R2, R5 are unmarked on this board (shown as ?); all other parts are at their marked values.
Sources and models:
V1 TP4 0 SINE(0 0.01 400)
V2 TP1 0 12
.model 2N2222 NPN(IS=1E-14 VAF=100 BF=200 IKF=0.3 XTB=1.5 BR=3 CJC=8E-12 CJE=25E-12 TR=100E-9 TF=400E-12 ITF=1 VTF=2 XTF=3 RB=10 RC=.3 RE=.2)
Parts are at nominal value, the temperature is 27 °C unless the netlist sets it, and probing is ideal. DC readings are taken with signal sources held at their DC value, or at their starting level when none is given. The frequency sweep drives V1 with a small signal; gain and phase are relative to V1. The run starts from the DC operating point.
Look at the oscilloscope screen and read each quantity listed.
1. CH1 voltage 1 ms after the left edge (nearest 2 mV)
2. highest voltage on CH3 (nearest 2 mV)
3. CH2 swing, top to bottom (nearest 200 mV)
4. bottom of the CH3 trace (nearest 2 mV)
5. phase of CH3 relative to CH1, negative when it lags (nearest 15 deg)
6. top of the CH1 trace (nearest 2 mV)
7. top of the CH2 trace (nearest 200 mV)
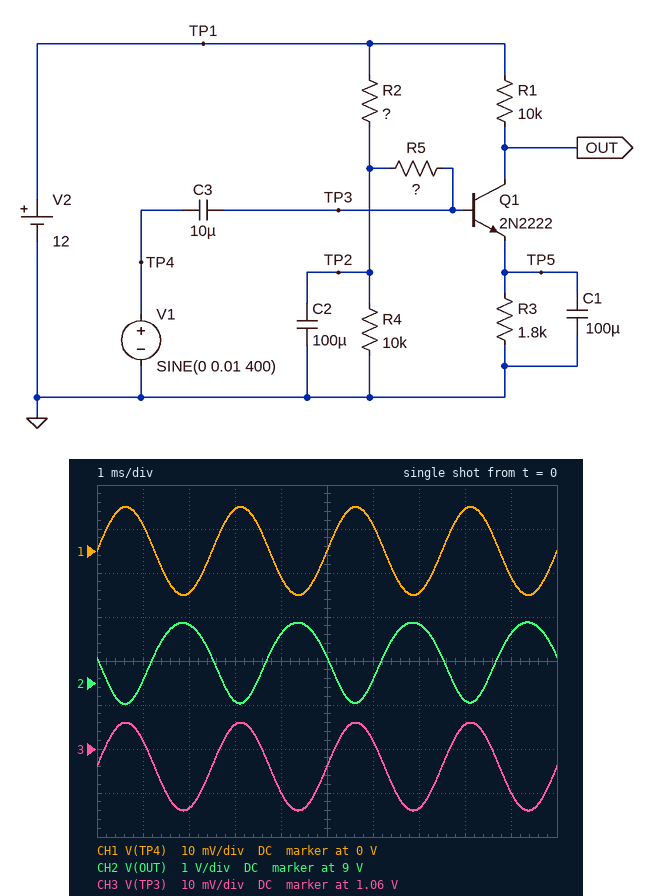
6 mV
1.066 V
1.8 V
1.046 V
0 deg
10 mV
10.4 V
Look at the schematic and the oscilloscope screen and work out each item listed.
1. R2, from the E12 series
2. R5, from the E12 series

100 kΩ
22 kΩ
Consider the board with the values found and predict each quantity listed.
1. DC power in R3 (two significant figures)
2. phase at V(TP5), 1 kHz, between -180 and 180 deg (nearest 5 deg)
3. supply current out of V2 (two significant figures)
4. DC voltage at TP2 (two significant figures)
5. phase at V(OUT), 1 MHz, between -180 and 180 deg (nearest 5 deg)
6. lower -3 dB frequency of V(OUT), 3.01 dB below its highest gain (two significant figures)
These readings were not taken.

110 µW
-90 deg
350 µA
1.1 V
165 deg
16 Hz
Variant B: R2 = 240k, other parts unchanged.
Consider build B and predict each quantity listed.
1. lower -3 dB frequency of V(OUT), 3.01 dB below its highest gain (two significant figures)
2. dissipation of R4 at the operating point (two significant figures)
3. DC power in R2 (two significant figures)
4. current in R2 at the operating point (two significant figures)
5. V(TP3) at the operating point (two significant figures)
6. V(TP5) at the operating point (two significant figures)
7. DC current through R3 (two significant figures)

3.7 MHz
23 µW
550 µW
48 µA
480 mV
2.1 mV
1.2 µA
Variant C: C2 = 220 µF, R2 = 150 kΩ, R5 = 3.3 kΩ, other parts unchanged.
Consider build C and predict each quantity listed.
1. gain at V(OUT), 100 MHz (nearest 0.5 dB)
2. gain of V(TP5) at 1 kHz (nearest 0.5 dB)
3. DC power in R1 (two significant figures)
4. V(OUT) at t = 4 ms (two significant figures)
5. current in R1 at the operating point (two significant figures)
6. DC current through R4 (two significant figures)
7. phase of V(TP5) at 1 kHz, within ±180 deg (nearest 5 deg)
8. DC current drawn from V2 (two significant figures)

5.0 dB
-45.5 dB
74 µW
11 V
86 µA
75 µA
-90 deg
160 µA
